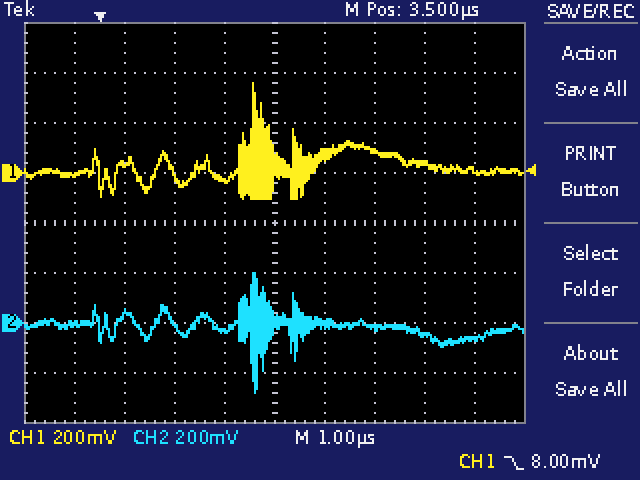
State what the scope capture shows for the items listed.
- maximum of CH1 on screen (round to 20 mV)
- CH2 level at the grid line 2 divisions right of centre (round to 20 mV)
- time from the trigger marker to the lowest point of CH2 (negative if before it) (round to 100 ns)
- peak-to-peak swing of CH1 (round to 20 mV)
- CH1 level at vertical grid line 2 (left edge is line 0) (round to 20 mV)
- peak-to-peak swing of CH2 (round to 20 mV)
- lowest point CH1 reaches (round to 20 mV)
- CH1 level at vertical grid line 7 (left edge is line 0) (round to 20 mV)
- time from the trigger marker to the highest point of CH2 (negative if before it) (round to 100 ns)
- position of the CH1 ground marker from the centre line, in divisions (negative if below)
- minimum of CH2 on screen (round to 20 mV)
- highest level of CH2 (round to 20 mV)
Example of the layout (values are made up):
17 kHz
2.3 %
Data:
360 mV
-20 mV
+3.1 µs
460 mV
40 mV
480 mV
-100 mV
80 mV
+3.1 µs
+1.0 div
-280 mV
200 mV
